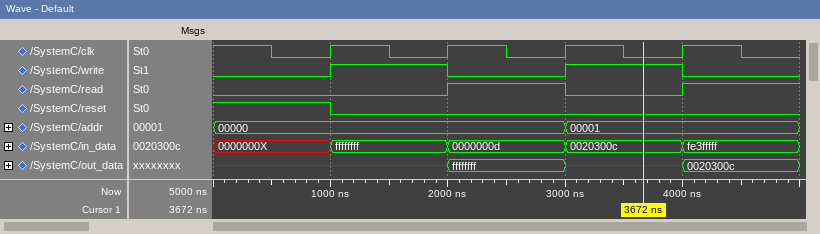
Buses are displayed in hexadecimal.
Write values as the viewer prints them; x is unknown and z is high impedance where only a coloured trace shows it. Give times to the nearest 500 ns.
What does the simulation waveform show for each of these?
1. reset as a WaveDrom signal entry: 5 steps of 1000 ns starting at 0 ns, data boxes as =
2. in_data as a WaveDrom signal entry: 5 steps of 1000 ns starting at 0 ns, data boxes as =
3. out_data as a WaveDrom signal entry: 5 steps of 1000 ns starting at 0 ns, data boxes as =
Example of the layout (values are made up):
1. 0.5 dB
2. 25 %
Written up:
1. {name: 'reset', wave: '10...'}
2. {name: 'in_data', wave: '=====', data: '0000000X ffffffff 0000000d 0020300c fe3fffff'}
3. {name: 'out_data', wave: 'x.=x=', data: 'ffffffff 0020300c'}
